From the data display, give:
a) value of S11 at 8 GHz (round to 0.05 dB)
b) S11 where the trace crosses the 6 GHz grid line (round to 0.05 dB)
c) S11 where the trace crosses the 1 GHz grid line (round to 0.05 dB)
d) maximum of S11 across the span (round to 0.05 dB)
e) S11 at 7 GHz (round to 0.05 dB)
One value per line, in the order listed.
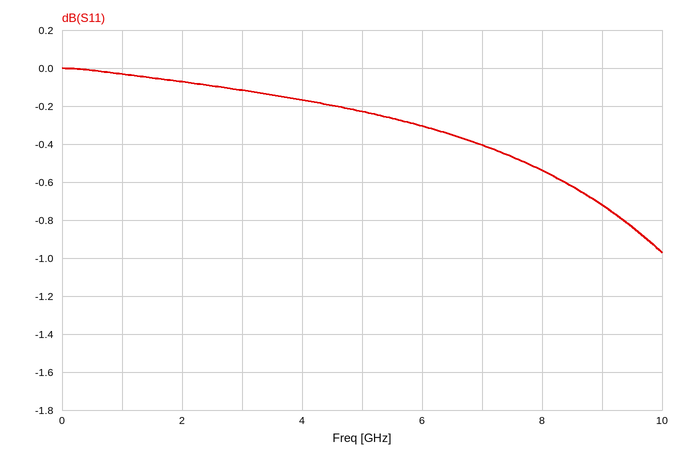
-0.55 dB
-0.30 dB
-0.05 dB
0.00 dB
-0.40 dB
